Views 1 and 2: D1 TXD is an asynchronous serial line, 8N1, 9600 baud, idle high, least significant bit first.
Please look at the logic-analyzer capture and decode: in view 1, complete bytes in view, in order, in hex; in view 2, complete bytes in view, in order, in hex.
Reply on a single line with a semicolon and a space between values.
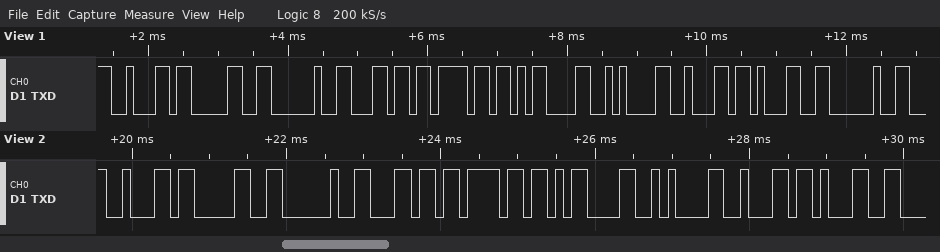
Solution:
0x62 0x30 0x20 0x6C 0x6F 0x0D 0x0A 0x62 0x31 0x20; 62 30 20 6C 6F 0D 0A 62 31
